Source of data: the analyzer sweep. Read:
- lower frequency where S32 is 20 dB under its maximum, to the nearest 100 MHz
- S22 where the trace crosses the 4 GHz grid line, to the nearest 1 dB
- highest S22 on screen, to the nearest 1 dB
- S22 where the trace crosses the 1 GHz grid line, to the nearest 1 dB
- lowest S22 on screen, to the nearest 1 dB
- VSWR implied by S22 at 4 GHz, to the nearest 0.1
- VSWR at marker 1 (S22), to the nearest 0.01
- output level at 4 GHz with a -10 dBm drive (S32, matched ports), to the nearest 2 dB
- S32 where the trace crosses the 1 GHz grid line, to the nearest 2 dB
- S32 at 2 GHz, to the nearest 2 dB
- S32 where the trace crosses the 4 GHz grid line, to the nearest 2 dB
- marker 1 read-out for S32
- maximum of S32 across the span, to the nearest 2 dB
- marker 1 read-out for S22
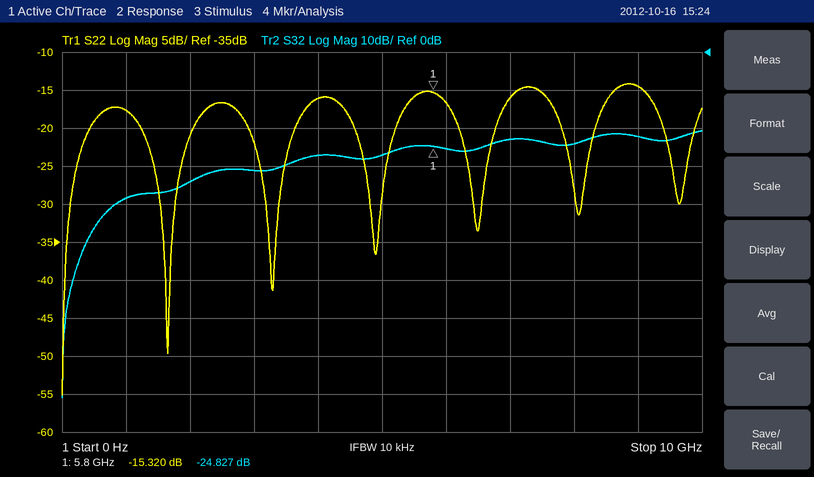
800 MHz
-16 dB
-14 dB
-18 dB
-55 dB
1.4
1.41
-38 dBm
-38 dB
-34 dB
-28 dB
-24.827 dB
-20 dB
-15.320 dB
